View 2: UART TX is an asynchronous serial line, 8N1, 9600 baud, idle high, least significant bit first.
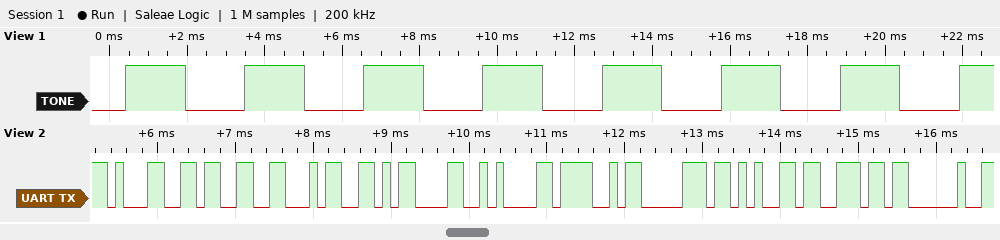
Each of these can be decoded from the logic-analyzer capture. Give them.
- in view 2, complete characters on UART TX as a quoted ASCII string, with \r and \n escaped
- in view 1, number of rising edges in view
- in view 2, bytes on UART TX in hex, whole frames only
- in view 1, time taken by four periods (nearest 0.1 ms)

"134\r\nOpen "
8
31 33 34 0D 0A 4F 70 65 6E 20
12.3 ms
